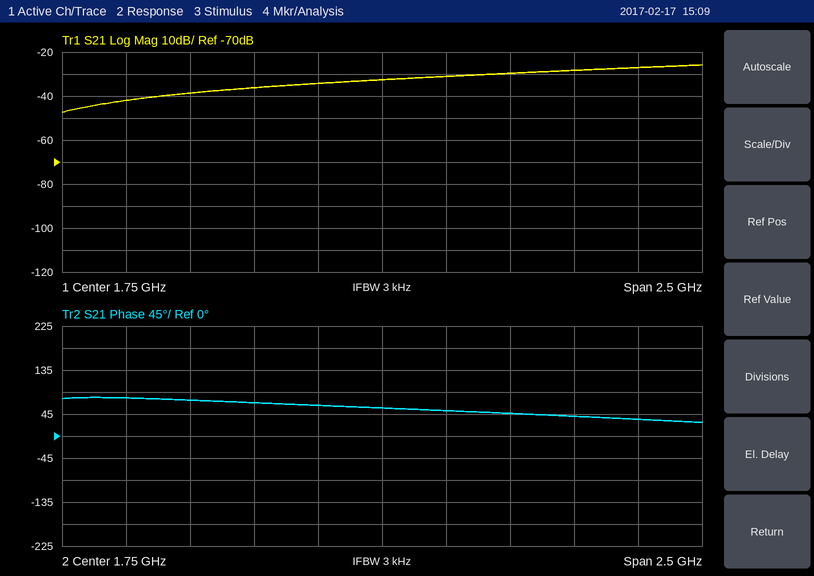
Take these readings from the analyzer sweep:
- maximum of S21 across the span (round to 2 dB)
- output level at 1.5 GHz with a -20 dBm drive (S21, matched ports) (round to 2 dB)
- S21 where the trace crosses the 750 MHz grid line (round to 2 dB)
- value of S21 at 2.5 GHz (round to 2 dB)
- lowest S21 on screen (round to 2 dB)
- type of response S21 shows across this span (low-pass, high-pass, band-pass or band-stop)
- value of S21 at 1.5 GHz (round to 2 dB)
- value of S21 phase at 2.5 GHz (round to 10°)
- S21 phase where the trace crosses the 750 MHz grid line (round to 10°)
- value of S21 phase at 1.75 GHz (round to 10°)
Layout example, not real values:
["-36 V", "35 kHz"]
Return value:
["-26 dB", "-54 dBm", "-42 dB", "-28 dB", "-48 dB", "high-pass", "-34 dB", "40°", "80°", "60°"]
